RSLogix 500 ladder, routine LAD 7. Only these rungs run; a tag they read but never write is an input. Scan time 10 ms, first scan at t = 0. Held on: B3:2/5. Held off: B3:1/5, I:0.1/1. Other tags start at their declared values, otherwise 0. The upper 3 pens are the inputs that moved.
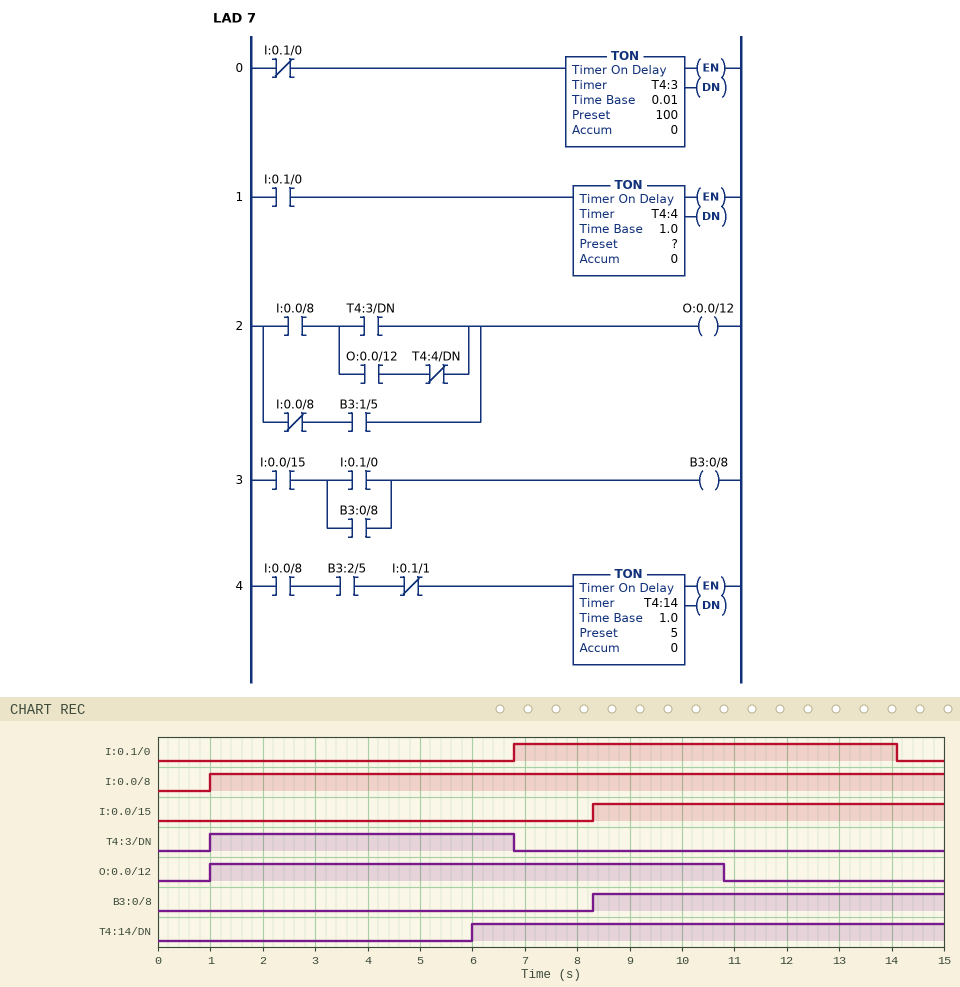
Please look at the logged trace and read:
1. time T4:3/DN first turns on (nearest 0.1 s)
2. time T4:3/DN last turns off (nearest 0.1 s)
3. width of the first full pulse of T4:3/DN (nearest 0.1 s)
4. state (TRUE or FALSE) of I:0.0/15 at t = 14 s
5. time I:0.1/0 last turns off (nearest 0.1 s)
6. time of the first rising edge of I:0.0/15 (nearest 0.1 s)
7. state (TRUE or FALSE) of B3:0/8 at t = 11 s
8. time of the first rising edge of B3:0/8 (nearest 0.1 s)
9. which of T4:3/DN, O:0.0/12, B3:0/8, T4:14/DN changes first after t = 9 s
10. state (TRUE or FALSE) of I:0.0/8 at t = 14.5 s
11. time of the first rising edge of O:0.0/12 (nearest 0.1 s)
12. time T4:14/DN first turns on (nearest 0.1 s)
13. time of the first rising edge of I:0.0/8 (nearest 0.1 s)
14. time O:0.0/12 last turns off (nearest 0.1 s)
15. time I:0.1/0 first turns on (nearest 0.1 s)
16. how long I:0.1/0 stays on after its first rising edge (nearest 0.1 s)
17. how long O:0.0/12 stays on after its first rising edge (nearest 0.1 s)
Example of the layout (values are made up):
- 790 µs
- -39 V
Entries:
- 1.0 s
- 6.8 s
- 5.8 s
- TRUE
- 14.1 s
- 8.3 s
- TRUE
- 8.3 s
- O:0.0/12
- TRUE
- 1.0 s
- 6.0 s
- 1.0 s
- 10.8 s
- 6.8 s
- 7.3 s
- 9.8 s
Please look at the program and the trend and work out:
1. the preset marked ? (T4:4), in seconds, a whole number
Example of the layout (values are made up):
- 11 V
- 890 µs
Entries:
- 4 s
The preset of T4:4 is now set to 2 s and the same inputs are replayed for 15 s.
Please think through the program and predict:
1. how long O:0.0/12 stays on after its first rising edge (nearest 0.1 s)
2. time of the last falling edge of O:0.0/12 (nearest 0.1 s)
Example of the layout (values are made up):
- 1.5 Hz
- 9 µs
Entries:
- 7.8 s
- 8.8 s
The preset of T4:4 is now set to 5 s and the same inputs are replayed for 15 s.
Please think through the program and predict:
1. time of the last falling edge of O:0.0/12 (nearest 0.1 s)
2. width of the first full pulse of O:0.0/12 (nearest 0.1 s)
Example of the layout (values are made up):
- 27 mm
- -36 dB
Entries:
- 11.8 s
- 10.8 s
